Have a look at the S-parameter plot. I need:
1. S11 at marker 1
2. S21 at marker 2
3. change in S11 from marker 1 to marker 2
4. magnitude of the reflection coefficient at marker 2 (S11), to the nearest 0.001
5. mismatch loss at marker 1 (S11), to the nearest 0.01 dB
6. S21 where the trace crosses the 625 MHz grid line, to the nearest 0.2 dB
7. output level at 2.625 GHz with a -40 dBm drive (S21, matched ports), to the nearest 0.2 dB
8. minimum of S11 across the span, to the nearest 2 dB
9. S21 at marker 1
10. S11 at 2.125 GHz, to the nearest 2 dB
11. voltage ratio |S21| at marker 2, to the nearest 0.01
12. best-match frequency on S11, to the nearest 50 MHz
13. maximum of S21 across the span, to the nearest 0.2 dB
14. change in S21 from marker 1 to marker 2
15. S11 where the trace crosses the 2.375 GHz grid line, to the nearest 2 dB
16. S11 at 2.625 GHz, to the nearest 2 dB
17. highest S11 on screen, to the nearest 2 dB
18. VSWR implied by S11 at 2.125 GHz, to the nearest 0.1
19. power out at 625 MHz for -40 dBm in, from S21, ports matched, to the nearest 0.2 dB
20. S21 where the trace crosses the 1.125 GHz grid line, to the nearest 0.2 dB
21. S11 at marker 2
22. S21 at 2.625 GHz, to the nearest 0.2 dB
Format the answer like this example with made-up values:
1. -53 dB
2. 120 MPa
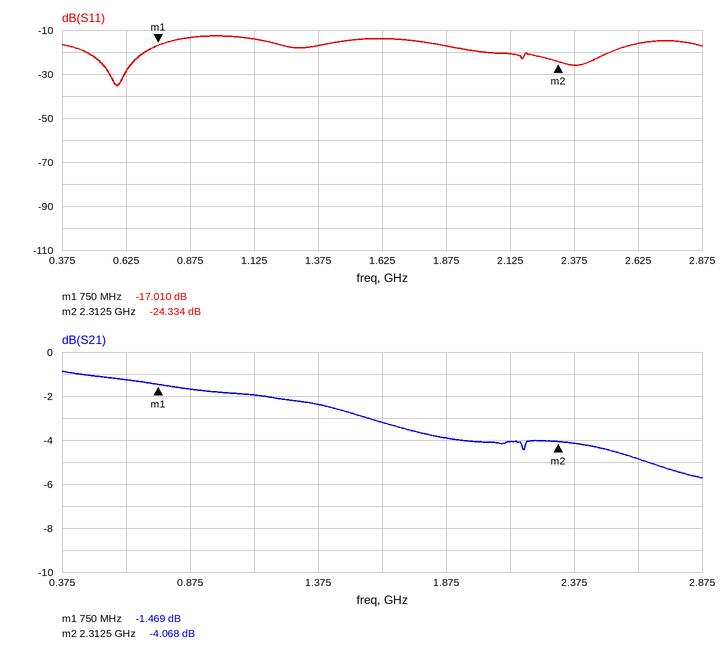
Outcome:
1. -17.010 dB
2. -4.068 dB
3. -7.324 dB
4. 0.061
5. 0.09 dB
6. -1.2 dB
7. -44.8 dBm
8. -36 dB
9. -1.469 dB
10. -20 dB
11. 0.63
12. 600 MHz
13. -0.8 dB
14. -2.599 dB
15. -26 dB
16. -16 dB
17. -12 dB
18. 1.2
19. -41.2 dBm
20. -2.0 dB
21. -24.334 dB
22. -4.8 dB
